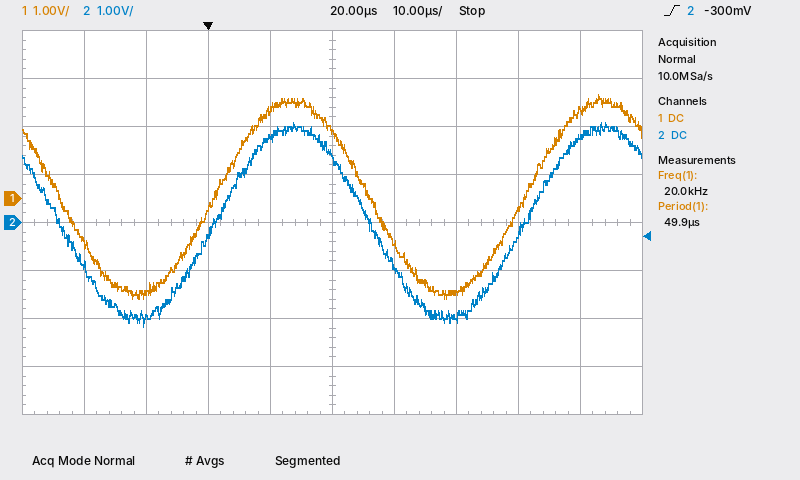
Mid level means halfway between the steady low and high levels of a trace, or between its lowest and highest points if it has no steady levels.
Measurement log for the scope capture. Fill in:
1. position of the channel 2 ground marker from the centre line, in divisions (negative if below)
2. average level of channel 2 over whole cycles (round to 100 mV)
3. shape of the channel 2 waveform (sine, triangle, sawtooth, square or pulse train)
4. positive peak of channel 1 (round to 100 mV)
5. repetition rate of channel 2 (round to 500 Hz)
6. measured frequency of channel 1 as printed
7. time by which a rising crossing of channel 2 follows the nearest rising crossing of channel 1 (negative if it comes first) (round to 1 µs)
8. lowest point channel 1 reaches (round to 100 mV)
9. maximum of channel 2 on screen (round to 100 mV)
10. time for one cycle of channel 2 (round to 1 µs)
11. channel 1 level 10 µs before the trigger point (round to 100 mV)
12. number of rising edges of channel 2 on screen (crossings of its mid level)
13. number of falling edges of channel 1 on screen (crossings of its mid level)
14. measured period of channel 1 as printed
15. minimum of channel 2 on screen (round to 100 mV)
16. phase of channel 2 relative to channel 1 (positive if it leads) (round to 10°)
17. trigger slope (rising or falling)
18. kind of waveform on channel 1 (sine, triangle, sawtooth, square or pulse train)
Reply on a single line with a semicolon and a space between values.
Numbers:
0.0 div; 0.0 V; sine; 2.2 V; 20.0 kHz; 20.0 kHz; 0 µs; -2.1 V; 2.1 V; 50 µs; -2.0 V; 2; 2; 49.9 µs; -2.2 V; 0°; rising; sine
